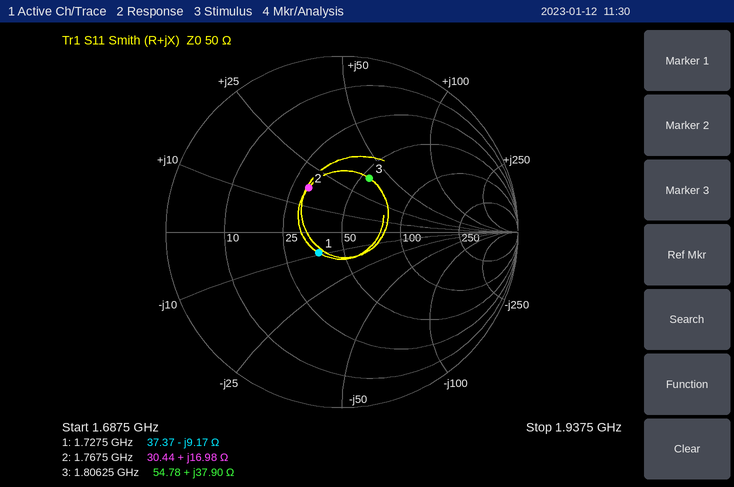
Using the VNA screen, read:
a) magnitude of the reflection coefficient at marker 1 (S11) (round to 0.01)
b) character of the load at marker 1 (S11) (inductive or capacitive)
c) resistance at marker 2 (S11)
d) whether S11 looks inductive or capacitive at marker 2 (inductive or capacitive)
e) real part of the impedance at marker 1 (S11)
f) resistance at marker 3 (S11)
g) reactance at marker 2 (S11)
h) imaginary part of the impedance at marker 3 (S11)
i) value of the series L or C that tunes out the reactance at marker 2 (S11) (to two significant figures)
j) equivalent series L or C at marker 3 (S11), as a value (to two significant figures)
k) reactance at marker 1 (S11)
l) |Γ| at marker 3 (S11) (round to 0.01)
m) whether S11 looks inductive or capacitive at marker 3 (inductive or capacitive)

0.18
capacitive
30.44 Ω
inductive
37.37 Ω
54.78 Ω
+16.98 Ω
+37.90 Ω
5.3 pF
3.3 nH
-9.17 Ω
0.34
inductive
